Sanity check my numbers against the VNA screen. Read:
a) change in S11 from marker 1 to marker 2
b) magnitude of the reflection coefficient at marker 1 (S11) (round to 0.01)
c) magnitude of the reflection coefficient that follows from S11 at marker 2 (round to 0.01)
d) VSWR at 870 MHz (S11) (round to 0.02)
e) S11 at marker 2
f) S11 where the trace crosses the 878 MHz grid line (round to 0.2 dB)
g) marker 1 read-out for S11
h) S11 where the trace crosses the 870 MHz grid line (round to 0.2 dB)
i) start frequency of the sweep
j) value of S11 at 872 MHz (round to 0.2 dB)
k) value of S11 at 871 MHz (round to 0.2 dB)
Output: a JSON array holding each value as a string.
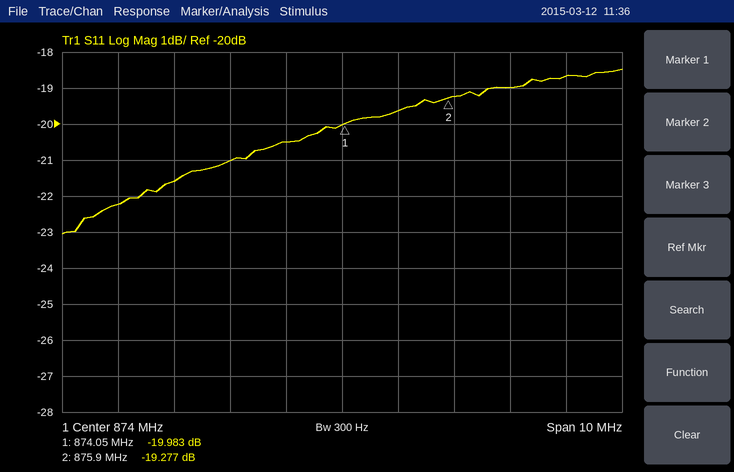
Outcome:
["0.706 dB", "0.10", "0.11", "1.16", "-19.277 dB", "-18.6 dB", "-19.983 dB", "-22.2 dB", "869 MHz", "-21.0 dB", "-21.6 dB"]
